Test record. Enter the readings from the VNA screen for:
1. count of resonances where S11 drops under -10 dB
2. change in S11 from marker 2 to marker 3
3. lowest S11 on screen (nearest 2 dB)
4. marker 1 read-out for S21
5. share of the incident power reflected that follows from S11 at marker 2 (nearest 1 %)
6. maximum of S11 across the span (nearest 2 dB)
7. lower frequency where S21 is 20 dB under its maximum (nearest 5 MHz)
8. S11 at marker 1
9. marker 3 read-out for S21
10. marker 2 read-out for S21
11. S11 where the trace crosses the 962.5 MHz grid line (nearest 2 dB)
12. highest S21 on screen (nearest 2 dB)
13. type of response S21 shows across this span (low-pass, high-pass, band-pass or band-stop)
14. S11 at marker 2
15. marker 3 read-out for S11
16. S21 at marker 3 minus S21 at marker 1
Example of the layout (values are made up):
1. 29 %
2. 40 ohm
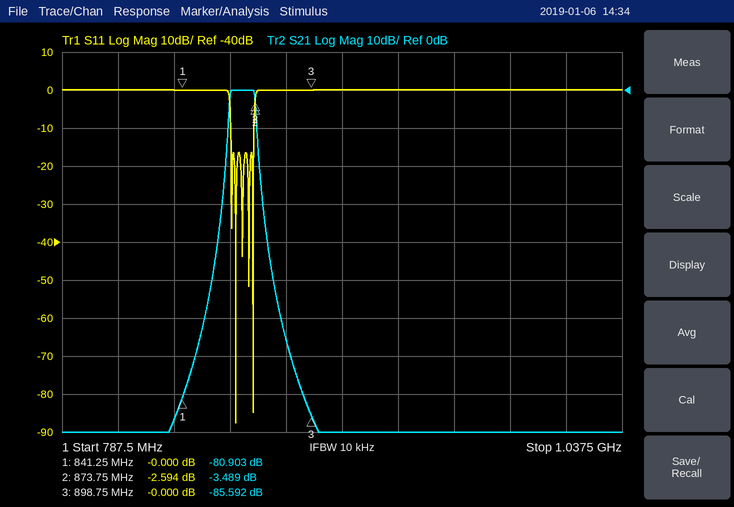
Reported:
1. 5
2. 2.594 dB
3. -88 dB
4. -80.903 dB
5. 55 %
6. 0 dB
7. 860 MHz
8. -0.000 dB
9. -85.592 dB
10. -3.489 dB
11. 0 dB
12. 0 dB
13. band-pass
14. -2.594 dB
15. -0.000 dB
16. -4.689 dB
